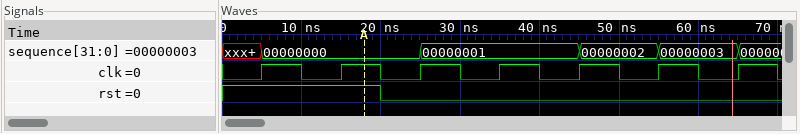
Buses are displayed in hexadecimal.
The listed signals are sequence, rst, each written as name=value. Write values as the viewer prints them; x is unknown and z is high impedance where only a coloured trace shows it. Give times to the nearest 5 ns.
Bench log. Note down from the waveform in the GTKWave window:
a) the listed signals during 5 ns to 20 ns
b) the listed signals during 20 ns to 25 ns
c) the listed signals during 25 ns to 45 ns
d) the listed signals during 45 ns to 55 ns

sequence=00000000, rst=1
sequence=00000000, rst=0
sequence=00000001, rst=0
sequence=00000002, rst=0
